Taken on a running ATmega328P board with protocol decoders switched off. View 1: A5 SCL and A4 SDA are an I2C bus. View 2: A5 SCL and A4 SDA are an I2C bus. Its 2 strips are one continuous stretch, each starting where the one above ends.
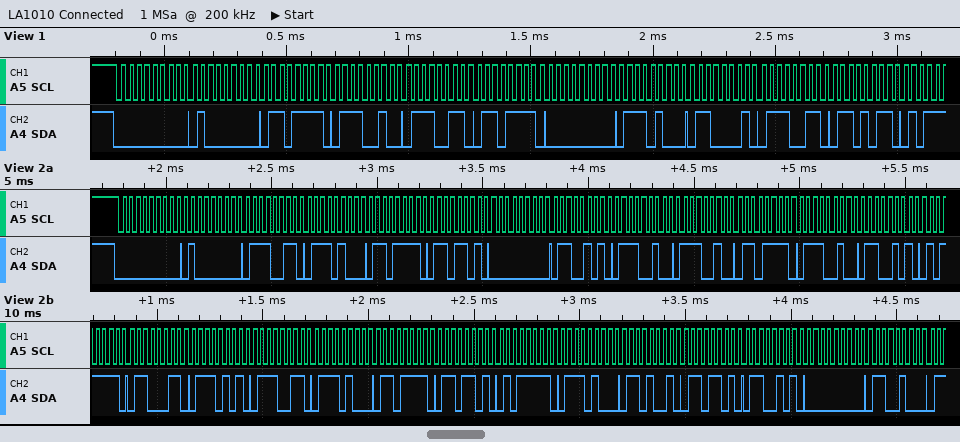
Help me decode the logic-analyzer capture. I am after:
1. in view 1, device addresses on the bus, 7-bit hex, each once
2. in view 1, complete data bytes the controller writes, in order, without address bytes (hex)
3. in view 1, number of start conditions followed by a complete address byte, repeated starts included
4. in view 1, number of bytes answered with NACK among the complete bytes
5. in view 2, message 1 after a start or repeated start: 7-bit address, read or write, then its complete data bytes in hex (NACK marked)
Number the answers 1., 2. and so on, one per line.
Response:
1. 0x00
2. 40 6F 72 73 6F 00 74 61 73 6B
3. 1
4. 0
5. 0x00 write: 40 73 74 6F 6D 00 65 72 72 6F 72 65 5F 63 75 73 74 6F 6D 5F 74 69 6D 65 00 64
